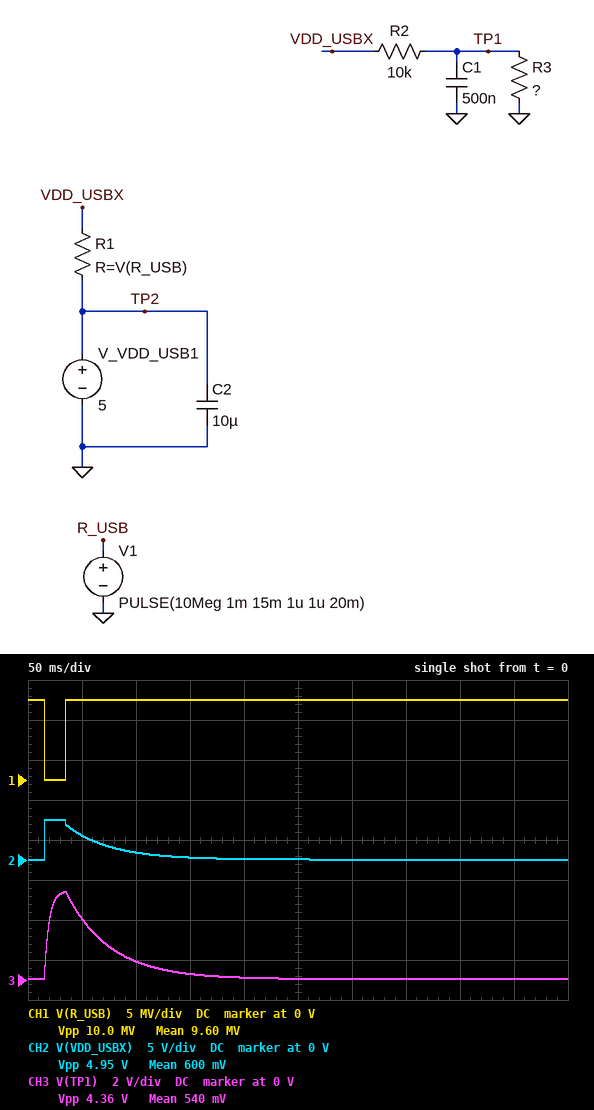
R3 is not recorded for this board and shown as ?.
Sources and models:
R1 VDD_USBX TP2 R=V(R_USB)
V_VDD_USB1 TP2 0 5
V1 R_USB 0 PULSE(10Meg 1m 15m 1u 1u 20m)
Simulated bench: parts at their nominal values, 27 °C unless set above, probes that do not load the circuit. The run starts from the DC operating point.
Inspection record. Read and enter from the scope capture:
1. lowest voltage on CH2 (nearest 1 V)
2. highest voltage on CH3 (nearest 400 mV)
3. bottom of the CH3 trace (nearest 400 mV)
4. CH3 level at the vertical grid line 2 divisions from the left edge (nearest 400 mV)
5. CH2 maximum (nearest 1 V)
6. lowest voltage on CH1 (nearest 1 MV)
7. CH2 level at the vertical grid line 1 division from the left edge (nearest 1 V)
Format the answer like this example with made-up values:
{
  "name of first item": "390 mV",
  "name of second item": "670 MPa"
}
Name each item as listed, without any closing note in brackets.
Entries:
{
  "lowest voltage on CH2": "0 V",
  "highest voltage on CH3": "4.4 V",
  "bottom of the CH3 trace": "0 V",
  "CH3 level at the vertical grid line 2 divisions from the left edge": "800 mV",
  "CH2 maximum": "5 V",
  "lowest voltage on CH1": "0 V",
  "CH2 level at the vertical grid line 1 division from the left edge": "3 V"
}
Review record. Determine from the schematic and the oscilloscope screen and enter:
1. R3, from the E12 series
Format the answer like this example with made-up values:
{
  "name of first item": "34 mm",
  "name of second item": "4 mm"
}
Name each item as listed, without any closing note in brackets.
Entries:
{
  "R3, from the E12 series": "82 kΩ"
}
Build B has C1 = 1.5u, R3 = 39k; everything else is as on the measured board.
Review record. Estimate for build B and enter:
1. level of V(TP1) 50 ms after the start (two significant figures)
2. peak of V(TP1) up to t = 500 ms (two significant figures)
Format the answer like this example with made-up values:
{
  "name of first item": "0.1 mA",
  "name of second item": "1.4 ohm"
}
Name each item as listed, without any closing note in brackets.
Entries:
{
  "level of V(TP1) 50 ms after the start": "2.5 V",
  "peak of V(TP1) up to t = 500 ms": "3.2 V"
}
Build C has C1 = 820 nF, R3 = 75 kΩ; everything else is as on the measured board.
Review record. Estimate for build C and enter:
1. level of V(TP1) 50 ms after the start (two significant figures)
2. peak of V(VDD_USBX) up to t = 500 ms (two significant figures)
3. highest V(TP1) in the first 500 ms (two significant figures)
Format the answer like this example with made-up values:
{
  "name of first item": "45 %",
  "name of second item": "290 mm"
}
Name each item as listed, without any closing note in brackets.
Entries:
{
  "level of V(TP1) 50 ms after the start": "3.2 V",
  "peak of V(VDD_USBX) up to t = 500 ms": "5.0 V",
  "highest V(TP1) in the first 500 ms": "4.1 V"
}
